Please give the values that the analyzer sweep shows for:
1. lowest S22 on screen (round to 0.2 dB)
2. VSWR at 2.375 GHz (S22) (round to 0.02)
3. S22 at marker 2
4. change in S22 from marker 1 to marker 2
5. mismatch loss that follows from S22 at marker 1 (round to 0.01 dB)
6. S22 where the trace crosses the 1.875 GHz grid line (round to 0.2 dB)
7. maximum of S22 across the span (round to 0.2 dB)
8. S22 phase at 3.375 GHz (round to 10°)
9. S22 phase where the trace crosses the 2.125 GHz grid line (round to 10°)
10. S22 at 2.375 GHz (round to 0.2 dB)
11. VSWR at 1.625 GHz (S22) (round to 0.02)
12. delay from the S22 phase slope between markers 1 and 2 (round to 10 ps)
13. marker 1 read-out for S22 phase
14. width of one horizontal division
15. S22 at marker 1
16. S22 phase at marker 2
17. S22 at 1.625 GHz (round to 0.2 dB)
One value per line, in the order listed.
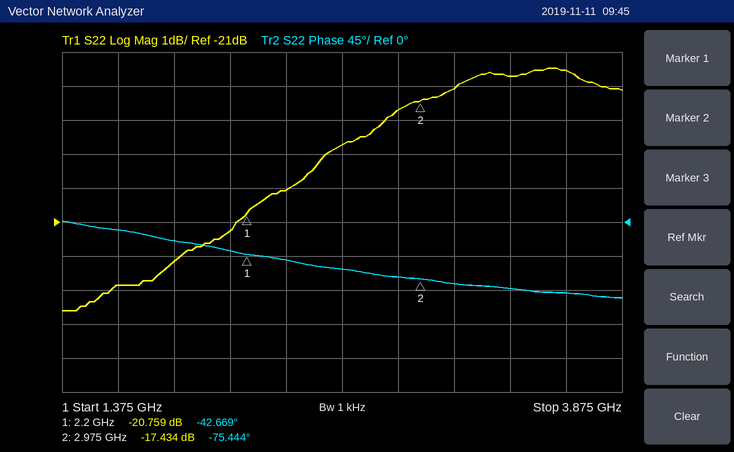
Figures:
-23.6 dB
1.22
-17.434 dB
3.325 dB
0.04 dB
-22.2 dB
-16.4 dB
-90°
-40°
-20.0 dB
1.16
120 ps
-42.669°
250 MHz
-20.759 dB
-75.444°
-22.8 dB
